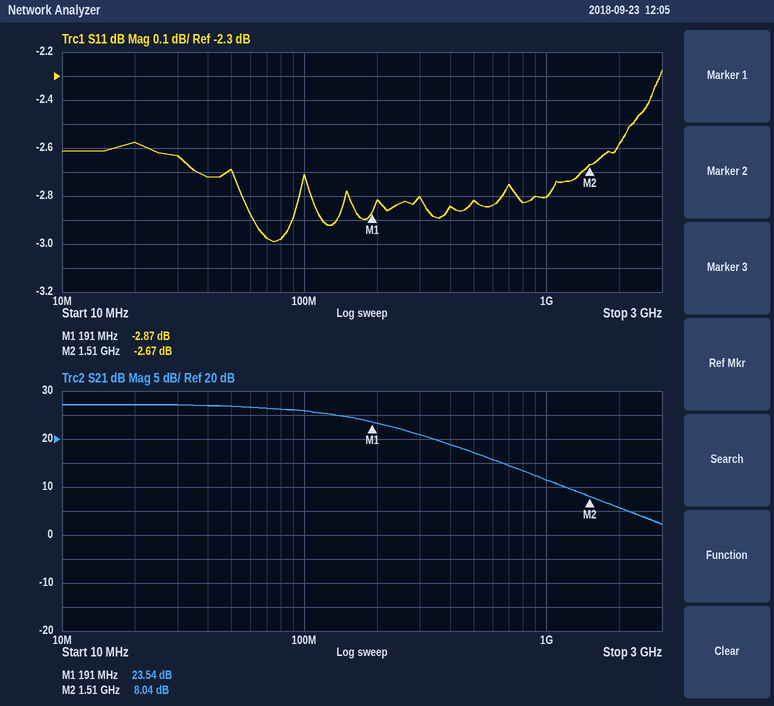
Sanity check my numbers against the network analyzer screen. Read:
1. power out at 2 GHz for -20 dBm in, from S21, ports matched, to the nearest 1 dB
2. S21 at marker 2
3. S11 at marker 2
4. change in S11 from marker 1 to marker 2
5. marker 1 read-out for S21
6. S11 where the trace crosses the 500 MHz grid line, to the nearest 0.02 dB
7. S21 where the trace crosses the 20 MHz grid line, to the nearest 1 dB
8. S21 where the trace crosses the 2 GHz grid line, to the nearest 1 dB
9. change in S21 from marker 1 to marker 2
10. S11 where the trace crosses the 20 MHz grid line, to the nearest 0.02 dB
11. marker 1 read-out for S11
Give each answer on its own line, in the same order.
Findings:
-14 dBm
8.04 dB
-2.67 dB
0.20 dB
23.54 dB
-2.82 dB
27 dB
6 dB
-15.50 dB
-2.58 dB
-2.87 dB
